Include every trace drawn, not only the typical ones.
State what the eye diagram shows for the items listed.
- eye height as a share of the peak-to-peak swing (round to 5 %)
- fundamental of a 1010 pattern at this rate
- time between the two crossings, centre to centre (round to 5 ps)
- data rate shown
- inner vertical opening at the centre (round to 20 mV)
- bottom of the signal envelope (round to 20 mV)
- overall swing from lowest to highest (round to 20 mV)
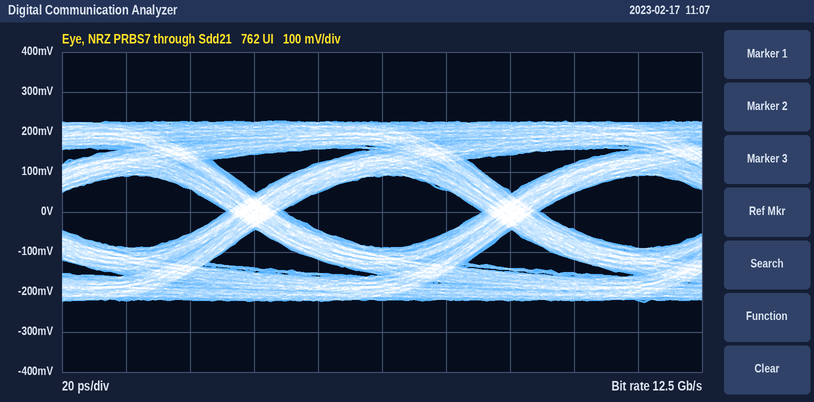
40 %
6.25 GHz
80 ps
12.5 Gb/s
180 mV
-220 mV
460 mV
